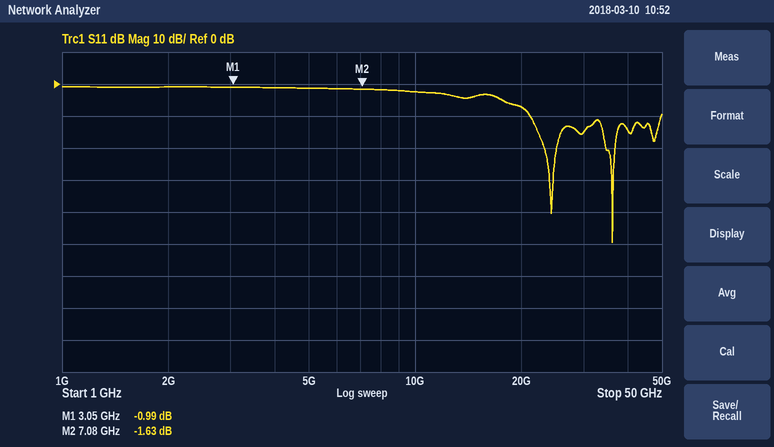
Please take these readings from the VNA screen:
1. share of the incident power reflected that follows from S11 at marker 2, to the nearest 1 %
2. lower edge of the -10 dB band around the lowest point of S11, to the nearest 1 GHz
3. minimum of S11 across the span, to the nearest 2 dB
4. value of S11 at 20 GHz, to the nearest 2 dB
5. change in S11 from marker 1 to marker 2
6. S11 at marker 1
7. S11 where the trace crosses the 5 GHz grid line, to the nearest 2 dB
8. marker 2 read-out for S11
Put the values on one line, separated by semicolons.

69 %; 21 GHz; -50 dB; -8 dB; -0.64 dB; -0.99 dB; -2 dB; -1.63 dB
